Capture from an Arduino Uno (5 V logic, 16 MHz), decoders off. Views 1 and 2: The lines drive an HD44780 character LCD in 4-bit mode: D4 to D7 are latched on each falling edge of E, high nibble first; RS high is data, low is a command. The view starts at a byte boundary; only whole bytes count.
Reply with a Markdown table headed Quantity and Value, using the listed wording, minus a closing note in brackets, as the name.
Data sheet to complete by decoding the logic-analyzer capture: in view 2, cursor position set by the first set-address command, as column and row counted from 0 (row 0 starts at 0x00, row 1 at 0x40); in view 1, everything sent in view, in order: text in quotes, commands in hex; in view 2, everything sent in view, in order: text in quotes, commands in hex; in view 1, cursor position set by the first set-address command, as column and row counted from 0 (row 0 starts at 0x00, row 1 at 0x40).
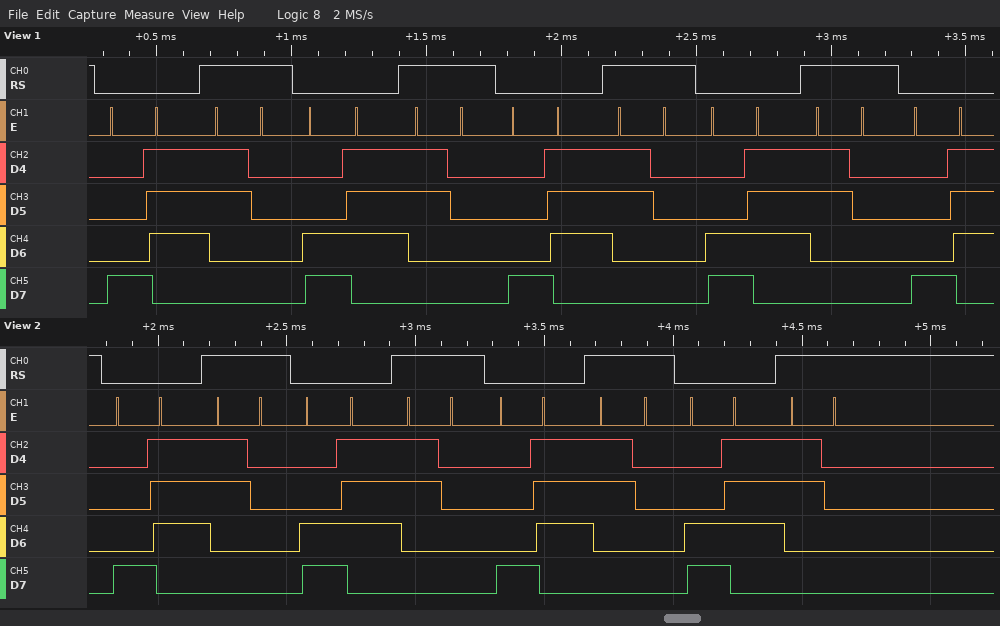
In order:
| Quantity | Value |
|---|---|
| in view 2, cursor position set by the first set-address command, as column and row counted from 0 | column 7, row 0 |
| in view 1, everything sent in view, in order: text in quotes, commands in hex | 0x87 "0" 0xC7 "0" 0x87 "0" 0xC7 "0" 0x87 |
| in view 2, everything sent in view, in order: text in quotes, commands in hex | 0x87 "0" 0xC7 "0" 0x87 "0" 0xC7 "0" |
| in view 1, cursor position set by the first set-address command, as column and row counted from 0 | column 7, row 0 |
